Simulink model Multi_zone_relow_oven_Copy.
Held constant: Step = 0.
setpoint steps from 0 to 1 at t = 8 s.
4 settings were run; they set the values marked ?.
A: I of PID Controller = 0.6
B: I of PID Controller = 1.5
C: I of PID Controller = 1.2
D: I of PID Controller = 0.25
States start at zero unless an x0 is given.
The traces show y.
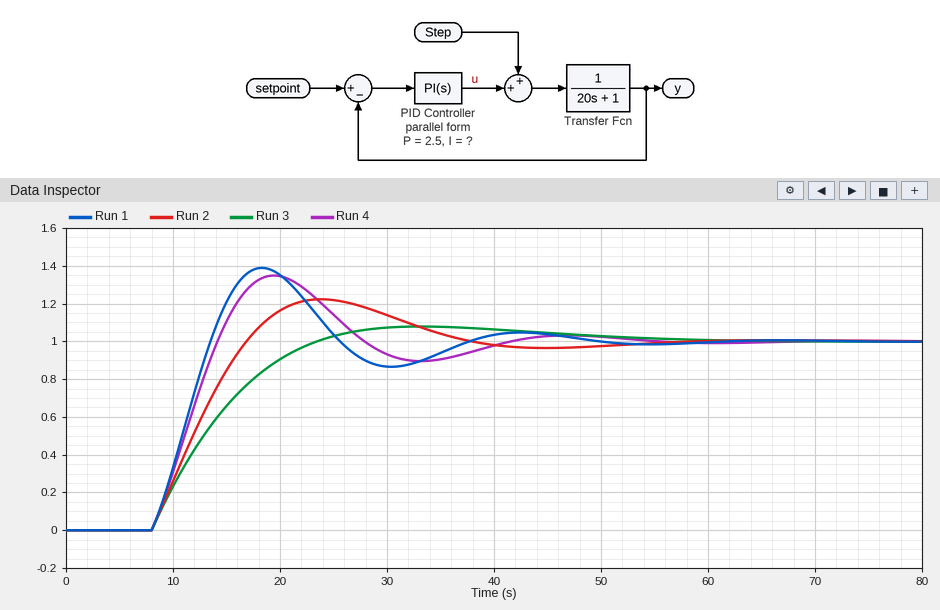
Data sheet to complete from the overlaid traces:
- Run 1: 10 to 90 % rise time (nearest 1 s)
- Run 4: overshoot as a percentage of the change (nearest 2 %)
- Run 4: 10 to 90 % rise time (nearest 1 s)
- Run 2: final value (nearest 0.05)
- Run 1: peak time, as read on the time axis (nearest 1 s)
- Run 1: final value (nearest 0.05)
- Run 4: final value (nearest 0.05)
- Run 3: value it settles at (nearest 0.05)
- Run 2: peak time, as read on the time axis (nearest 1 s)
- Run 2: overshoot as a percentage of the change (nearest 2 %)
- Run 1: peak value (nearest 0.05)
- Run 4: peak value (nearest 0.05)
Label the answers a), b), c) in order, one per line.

a) 4 s
b) 34 %
c) 5 s
d) 1.00
e) 18 s
f) 1.00
g) 1.00
h) 1.00
i) 24 s
j) 22 %
k) 1.40
l) 1.35
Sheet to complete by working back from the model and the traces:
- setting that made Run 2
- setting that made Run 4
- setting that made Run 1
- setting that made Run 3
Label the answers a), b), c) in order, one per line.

a) A
b) C
c) B
d) D
